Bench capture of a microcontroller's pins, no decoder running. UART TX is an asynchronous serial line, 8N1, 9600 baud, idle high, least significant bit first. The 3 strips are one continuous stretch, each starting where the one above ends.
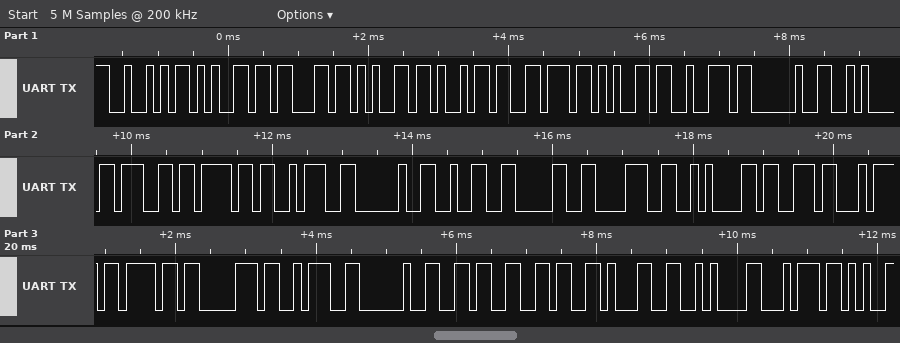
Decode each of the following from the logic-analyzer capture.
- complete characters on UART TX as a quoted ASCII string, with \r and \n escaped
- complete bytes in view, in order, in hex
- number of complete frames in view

"Receiver \ngo: 208\nstop: 661\nt"
52 65 63 65 69 76 65 72 20 0A 67 6F 3A 20 32 30 38 0A 73 74 6F 70 3A 20 36 36 31 0A 74
29
